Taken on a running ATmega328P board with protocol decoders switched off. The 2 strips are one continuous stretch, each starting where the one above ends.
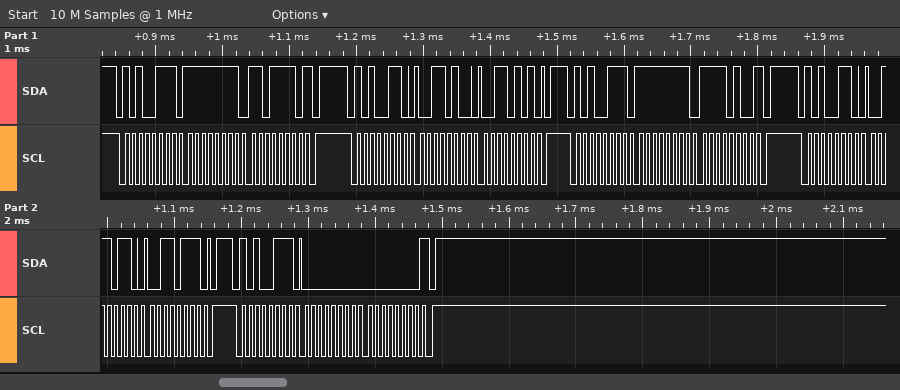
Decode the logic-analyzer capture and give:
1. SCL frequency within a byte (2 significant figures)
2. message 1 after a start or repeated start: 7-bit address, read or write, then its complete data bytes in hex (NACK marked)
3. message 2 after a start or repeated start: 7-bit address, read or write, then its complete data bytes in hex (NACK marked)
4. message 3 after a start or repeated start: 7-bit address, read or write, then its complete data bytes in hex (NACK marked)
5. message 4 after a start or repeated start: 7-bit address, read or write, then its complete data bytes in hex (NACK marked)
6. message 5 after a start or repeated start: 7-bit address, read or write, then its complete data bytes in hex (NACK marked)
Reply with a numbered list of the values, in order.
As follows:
1. 100 kHz
2. 0x53 read: FF DE NACK
3. 0x53 write: 34 35
4. 0x53 read: FF F4 NACK
5. 0x53 write: 36 37
6. 0x53 read: 00 00 NACK
